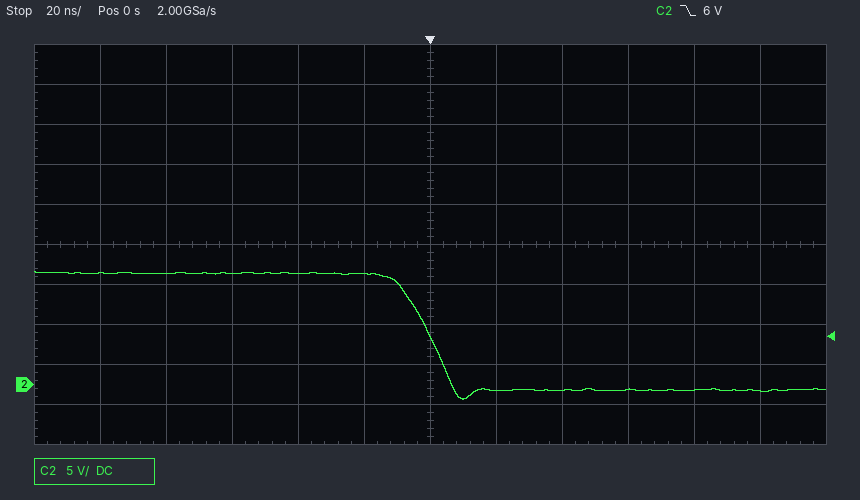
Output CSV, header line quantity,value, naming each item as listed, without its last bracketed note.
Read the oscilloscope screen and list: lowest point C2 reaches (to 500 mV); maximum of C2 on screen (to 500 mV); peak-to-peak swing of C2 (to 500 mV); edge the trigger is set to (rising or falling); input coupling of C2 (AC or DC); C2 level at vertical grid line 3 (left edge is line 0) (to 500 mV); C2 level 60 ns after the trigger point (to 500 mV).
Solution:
quantity,value
lowest point C2 reaches,-2.0 V
maximum of C2 on screen,14.0 V
peak-to-peak swing of C2,16.0 V
edge the trigger is set to,falling
input coupling of C2,DC
C2 level at vertical grid line 3 (left edge is line 0),14.0 V
C2 level 60 ns after the trigger point,-500 mV
